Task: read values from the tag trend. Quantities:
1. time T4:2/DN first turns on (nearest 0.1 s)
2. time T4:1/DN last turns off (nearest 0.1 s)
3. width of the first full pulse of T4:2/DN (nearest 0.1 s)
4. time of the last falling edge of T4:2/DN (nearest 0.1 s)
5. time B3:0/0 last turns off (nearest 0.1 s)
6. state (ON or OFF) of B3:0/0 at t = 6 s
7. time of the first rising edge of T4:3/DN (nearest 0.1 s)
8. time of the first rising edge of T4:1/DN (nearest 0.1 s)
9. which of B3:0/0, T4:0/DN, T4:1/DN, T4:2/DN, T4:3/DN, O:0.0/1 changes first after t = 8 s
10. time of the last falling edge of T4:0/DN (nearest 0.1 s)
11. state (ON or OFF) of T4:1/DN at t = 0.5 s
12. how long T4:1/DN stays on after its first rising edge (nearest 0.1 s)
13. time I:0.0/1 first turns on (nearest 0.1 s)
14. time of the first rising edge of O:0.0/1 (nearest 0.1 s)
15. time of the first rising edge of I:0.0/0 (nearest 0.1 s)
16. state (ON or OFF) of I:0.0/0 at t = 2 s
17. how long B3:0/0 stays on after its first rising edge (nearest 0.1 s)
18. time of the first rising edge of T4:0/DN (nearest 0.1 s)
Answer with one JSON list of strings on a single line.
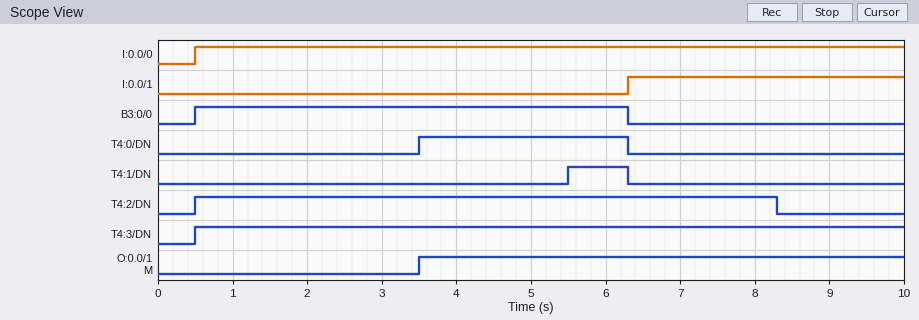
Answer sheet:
["0.5 s", "6.3 s", "7.8 s", "8.3 s", "6.3 s", "ON", "0.5 s", "5.5 s", "T4:2/DN", "6.3 s", "OFF", "0.8 s", "6.3 s", "3.5 s", "0.5 s", "ON", "5.8 s", "3.5 s"]
